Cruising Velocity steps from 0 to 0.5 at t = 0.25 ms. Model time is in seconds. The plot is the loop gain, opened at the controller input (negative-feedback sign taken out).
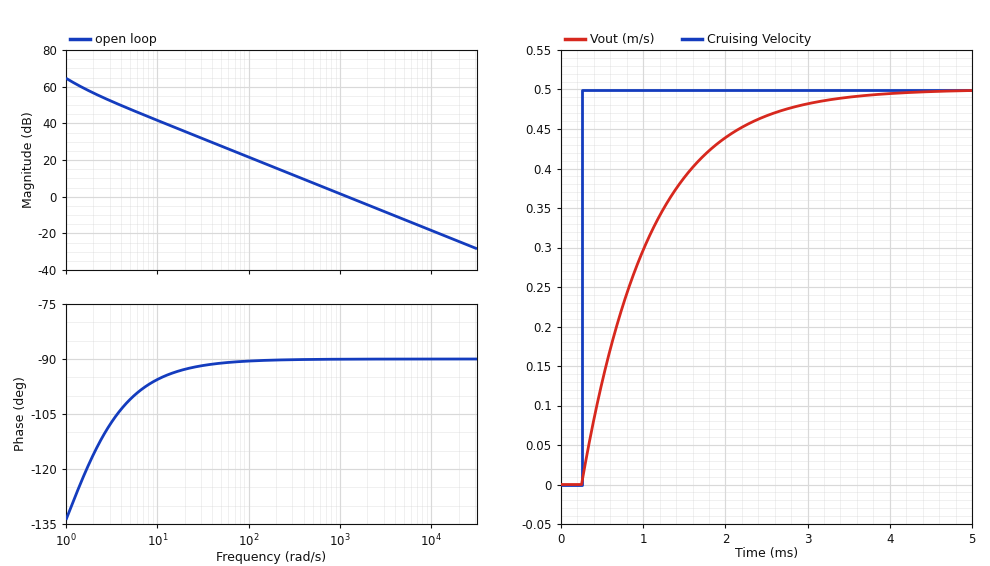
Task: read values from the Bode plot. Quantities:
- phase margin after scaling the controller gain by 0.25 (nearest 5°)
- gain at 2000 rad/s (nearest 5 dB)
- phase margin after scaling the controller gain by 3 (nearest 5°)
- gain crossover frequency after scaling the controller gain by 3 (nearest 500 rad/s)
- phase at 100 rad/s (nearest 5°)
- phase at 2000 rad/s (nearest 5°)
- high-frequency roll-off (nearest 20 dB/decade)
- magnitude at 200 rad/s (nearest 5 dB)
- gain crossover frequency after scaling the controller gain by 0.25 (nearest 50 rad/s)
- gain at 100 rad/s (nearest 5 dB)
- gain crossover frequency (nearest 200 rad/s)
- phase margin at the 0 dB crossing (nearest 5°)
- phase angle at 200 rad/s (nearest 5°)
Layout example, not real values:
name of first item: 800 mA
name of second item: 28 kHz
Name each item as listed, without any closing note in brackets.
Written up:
phase margin after scaling the controller gain by 0.25: 90°
gain at 2000 rad/s: -5 dB
phase margin after scaling the controller gain by 3: 90°
gain crossover frequency after scaling the controller gain by 3: 3500 rad/s
phase at 100 rad/s: -90°
phase at 2000 rad/s: -90°
high-frequency roll-off: -20 dB/decade
magnitude at 200 rad/s: 15 dB
gain crossover frequency after scaling the controller gain by 0.25: 300 rad/s
gain at 100 rad/s: 20 dB
gain crossover frequency: 1200 rad/s
phase margin at the 0 dB crossing: 90°
phase angle at 200 rad/s: -90°
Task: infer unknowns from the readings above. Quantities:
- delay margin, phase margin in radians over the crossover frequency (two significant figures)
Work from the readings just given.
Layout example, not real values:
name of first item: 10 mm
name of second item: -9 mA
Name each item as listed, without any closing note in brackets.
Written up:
delay margin, phase margin in radians over the crossover frequency: 0.0013 s
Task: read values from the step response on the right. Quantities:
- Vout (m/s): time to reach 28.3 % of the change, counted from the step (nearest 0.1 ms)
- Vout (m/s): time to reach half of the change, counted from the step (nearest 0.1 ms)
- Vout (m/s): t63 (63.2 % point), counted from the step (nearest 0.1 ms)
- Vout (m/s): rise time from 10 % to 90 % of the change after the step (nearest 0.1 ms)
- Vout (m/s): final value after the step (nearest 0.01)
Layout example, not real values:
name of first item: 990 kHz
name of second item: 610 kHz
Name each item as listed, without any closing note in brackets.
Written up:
Vout (m/s): time to reach 28.3 % of the change, counted from the step: 0.3 ms
Vout (m/s): time to reach half of the change, counted from the step: 0.6 ms
Vout (m/s): t63 (63.2 % point), counted from the step: 0.8 ms
Vout (m/s): rise time from 10 % to 90 % of the change after the step: 1.8 ms
Vout (m/s): final value after the step: 0.50
